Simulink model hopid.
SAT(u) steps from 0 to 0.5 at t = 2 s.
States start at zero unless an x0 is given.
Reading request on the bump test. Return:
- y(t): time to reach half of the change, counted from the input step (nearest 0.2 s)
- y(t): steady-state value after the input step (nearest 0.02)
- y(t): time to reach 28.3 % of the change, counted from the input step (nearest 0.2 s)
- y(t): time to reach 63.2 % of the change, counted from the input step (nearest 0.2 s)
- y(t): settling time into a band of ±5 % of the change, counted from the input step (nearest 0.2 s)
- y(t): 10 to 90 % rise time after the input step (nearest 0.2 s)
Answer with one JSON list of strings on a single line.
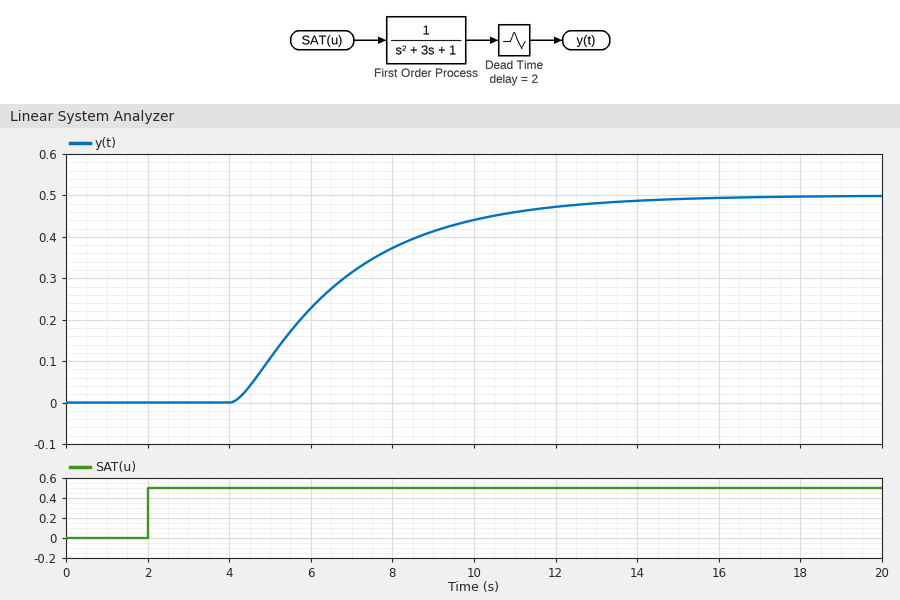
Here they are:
["4.2 s", "0.50", "3.2 s", "5.0 s", "10.2 s", "5.8 s"]
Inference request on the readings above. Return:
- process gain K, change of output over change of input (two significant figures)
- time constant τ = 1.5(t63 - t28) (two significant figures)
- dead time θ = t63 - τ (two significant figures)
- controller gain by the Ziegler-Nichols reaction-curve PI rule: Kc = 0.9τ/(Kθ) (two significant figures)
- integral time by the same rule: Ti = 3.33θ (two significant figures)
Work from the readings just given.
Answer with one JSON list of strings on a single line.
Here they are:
["1.0", "2.7 s", "2.3 s", "1.1", "7.7 s"]
